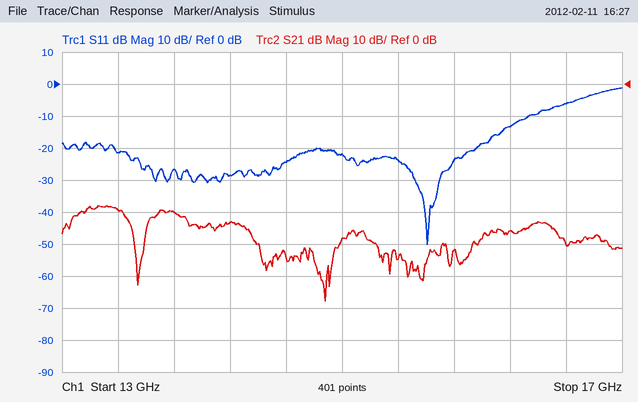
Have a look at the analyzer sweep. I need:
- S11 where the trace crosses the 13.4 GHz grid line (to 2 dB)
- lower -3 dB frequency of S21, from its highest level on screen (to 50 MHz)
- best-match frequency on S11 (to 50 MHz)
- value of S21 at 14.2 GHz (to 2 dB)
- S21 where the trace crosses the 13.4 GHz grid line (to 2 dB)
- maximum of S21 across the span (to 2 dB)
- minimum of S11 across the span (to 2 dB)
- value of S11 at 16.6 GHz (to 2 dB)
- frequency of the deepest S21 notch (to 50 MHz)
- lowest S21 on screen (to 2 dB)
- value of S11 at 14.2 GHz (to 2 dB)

-22 dB
13.10 GHz
15.60 GHz
-44 dB
-40 dB
-38 dB
-50 dB
-6 dB
14.90 GHz
-68 dB
-28 dB
